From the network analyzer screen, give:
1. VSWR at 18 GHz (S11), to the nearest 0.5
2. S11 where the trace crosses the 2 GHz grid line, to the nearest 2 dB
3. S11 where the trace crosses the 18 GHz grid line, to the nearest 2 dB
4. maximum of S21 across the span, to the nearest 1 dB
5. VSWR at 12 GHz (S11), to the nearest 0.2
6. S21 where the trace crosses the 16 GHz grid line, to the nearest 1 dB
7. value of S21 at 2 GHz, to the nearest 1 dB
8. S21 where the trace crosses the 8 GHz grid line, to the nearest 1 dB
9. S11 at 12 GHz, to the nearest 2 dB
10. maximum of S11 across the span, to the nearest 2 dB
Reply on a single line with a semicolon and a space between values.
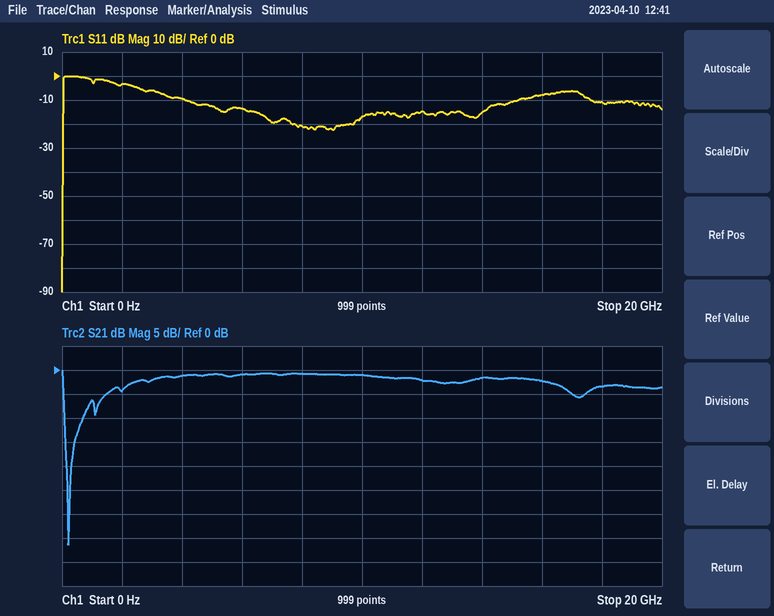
2.0; -4 dB; -10 dB; 0 dB; 1.4; -2 dB; -4 dB; -1 dB; -14 dB; 0 dB
